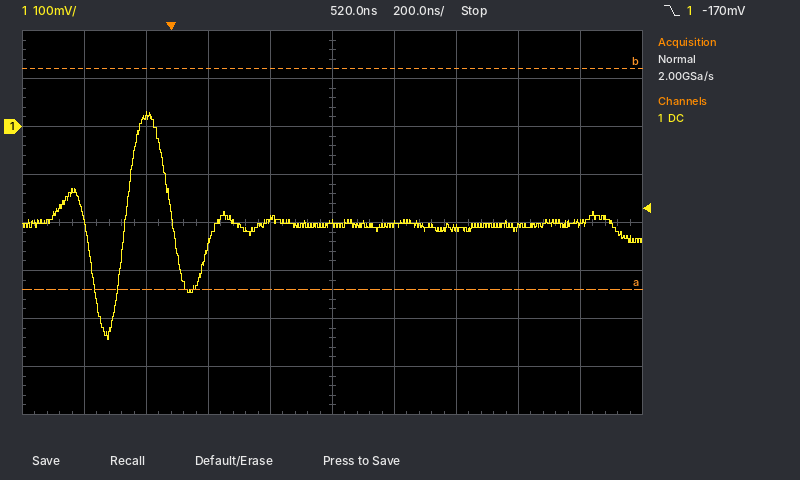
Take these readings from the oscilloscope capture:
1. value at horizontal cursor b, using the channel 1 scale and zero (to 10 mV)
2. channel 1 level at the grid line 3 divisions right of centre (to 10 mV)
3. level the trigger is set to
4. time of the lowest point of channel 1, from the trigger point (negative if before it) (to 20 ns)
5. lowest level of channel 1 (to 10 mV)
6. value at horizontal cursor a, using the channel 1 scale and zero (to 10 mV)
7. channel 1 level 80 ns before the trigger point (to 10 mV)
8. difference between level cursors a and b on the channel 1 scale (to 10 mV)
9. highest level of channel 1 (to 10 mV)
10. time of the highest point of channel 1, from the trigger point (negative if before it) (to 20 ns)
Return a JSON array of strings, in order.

["120 mV", "-210 mV", "-170 mV", "-200 ns", "-440 mV", "-340 mV", "20 mV", "460 mV", "30 mV", "-80 ns"]
